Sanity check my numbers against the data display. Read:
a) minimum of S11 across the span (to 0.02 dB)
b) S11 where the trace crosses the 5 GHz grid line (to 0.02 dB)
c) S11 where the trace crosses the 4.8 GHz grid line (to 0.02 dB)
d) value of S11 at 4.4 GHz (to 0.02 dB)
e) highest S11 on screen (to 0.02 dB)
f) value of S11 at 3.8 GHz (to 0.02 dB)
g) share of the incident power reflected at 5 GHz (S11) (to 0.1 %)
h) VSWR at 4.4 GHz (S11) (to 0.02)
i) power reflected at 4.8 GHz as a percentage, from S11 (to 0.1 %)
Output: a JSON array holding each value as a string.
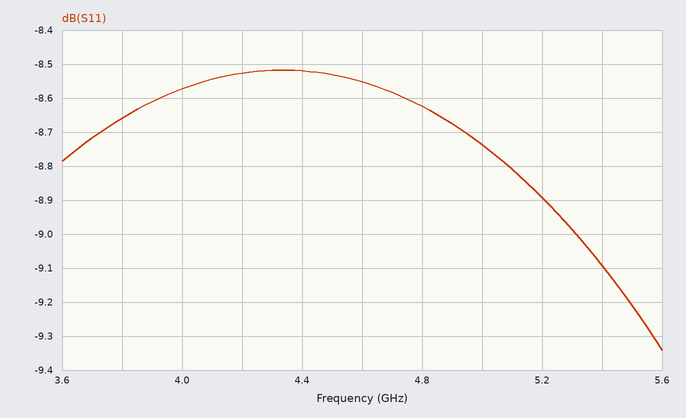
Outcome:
["-9.34 dB", "-8.74 dB", "-8.62 dB", "-8.52 dB", "-8.52 dB", "-8.66 dB", "13.4 %", "2.20", "13.7 %"]
